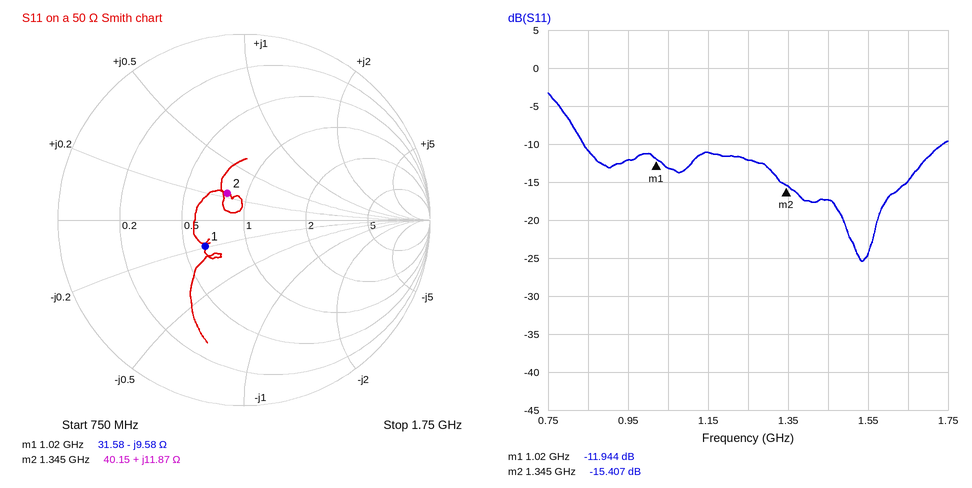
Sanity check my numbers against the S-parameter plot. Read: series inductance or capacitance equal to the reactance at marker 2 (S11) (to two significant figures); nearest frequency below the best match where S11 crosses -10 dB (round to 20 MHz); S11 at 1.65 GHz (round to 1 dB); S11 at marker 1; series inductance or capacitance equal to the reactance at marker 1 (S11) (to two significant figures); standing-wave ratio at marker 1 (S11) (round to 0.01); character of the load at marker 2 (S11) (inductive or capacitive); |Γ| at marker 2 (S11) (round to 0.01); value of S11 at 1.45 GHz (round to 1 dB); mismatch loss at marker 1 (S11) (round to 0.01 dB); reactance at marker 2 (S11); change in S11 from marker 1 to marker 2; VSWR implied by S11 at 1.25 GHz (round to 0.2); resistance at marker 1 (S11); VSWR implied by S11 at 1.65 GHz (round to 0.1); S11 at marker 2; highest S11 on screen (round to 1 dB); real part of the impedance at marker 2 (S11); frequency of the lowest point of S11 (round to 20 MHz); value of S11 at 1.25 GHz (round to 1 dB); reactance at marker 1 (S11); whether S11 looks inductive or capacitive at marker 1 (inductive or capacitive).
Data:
1.4 nH
840 MHz
-15 dB
-11.944 dB
16 pF
1.68
inductive
0.17
-17 dB
0.29 dB
+11.87 Ω
-3.463 dB
1.6
31.58 Ω
1.4
-15.407 dB
-3 dB
40.15 Ω
1.54 GHz
-12 dB
-9.58 Ω
capacitive
